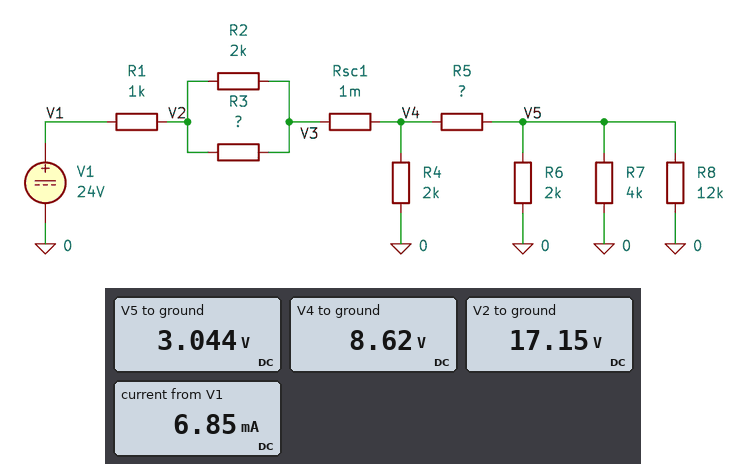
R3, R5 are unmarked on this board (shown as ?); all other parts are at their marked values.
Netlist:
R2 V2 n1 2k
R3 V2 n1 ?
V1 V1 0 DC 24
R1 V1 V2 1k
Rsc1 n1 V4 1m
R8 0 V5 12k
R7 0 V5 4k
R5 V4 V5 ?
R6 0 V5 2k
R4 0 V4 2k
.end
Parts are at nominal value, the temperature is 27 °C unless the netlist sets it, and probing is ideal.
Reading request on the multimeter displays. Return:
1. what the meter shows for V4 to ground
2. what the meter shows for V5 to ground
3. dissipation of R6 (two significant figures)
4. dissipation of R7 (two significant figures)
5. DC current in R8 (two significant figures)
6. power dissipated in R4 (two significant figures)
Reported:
8.62 V
3.044 V
4.6 mW
2.3 mW
250 µA
37 mW
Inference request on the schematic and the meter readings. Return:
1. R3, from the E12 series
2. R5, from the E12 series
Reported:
3.3 kΩ
2.2 kΩ
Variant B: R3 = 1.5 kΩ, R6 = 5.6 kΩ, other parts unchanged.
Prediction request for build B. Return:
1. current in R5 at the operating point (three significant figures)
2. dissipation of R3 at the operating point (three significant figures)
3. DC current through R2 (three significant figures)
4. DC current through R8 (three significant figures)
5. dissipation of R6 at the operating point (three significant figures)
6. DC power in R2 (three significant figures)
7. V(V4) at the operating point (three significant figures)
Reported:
2.43 mA
27.4 mW
3.21 mA
396 µA
4.03 mW
20.6 mW
10.1 V
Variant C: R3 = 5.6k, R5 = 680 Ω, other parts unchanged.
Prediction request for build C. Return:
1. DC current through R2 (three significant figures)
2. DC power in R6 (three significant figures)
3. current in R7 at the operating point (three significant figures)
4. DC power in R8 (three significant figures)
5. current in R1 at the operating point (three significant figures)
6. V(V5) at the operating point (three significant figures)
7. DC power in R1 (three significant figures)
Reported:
5.14 mA
9.30 mW
1.08 mA
1.55 mW
6.97 mA
4.31 V
48.6 mW
